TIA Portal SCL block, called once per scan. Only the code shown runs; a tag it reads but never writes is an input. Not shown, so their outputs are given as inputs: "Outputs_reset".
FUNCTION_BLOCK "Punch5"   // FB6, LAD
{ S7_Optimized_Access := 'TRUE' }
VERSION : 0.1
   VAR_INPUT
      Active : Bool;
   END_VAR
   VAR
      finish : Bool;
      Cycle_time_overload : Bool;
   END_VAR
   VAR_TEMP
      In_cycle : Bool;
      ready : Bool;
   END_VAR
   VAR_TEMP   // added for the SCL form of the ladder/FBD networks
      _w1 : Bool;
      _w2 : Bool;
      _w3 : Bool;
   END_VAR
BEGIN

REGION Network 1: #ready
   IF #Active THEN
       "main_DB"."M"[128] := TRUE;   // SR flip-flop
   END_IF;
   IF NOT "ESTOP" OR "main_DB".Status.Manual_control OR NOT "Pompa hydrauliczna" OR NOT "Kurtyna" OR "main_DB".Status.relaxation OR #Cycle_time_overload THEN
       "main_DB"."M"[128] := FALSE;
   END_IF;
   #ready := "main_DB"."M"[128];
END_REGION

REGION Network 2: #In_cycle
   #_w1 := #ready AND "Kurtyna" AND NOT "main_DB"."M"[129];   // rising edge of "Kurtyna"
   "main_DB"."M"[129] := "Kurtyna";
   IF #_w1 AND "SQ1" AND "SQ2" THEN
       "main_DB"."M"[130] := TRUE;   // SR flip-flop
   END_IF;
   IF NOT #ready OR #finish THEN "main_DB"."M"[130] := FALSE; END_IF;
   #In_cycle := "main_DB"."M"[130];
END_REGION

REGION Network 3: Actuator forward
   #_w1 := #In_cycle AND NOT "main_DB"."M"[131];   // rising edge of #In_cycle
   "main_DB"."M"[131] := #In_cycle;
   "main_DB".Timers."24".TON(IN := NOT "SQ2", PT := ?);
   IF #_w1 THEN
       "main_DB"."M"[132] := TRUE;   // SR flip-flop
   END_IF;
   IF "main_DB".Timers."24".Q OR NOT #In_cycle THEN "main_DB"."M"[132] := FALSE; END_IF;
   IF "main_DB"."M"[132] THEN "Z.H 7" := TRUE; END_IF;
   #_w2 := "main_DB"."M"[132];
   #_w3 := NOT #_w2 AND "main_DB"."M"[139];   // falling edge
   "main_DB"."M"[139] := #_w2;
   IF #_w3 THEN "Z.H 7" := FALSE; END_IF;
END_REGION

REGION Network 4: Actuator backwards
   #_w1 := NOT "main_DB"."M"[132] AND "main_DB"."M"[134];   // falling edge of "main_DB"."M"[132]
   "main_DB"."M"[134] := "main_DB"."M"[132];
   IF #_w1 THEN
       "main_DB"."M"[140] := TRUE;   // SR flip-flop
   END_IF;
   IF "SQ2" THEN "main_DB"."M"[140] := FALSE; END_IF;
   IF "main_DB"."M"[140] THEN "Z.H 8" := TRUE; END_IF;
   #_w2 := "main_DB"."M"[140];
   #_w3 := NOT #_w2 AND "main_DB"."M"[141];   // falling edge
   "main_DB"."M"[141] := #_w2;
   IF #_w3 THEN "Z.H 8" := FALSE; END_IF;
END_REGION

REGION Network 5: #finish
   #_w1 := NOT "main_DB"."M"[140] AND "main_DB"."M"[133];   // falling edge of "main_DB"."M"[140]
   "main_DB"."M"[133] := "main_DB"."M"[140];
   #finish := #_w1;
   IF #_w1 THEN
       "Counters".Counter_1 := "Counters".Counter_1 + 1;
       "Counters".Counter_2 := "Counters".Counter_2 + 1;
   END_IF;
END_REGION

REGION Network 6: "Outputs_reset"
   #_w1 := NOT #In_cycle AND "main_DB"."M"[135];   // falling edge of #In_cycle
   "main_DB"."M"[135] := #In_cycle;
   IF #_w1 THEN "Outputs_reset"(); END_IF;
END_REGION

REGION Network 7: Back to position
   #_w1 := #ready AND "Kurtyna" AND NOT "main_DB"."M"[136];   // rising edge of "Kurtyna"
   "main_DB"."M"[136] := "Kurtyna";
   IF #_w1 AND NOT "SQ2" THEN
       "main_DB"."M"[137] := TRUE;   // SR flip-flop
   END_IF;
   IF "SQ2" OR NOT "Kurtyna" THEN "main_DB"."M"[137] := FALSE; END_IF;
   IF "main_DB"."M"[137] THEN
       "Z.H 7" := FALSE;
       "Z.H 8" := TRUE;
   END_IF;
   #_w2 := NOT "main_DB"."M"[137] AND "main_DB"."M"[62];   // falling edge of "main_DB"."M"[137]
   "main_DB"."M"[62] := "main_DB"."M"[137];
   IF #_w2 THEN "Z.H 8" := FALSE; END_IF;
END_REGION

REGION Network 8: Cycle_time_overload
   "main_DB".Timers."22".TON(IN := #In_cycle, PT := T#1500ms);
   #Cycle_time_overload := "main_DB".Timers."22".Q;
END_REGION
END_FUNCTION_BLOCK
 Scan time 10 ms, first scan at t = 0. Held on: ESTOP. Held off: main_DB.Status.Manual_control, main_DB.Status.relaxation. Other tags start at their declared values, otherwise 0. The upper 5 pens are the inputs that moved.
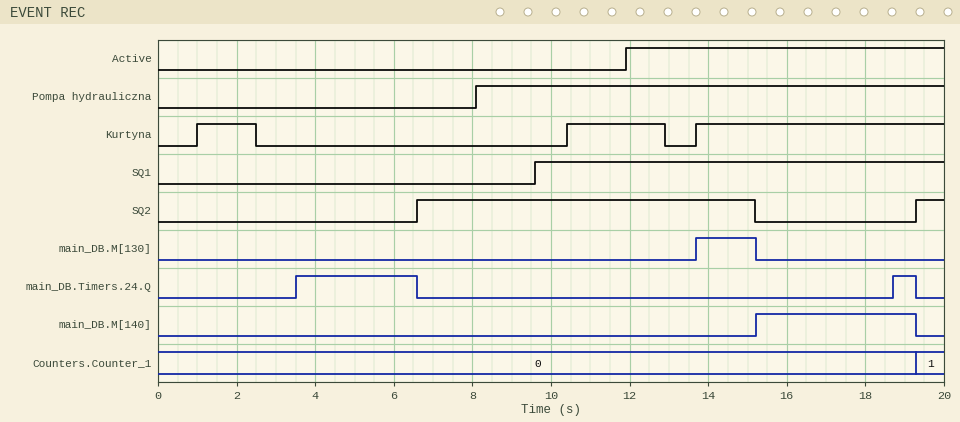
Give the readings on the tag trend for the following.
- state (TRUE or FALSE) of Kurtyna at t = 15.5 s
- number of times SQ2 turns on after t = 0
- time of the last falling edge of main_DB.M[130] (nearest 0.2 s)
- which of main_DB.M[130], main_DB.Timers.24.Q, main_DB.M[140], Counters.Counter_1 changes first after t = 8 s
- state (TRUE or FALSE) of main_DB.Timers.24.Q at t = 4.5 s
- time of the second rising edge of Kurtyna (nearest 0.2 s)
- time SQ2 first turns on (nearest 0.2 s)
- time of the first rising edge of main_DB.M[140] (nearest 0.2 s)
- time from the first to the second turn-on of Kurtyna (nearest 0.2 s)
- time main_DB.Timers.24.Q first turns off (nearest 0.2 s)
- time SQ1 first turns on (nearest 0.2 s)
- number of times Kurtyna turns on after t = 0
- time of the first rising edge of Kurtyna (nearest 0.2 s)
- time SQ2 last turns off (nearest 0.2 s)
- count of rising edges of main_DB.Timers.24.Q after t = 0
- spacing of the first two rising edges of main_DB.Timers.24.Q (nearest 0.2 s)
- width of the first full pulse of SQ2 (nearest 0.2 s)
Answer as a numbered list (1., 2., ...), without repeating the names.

1. TRUE
2. 2
3. 15.2 s
4. main_DB.M[130]
5. TRUE
6. 10.4 s
7. 6.6 s
8. 15.2 s
9. 9.4 s
10. 6.6 s
11. 9.6 s
12. 3
13. 1.0 s
14. 15.2 s
15. 2
16. 15.2 s
17. 8.6 s
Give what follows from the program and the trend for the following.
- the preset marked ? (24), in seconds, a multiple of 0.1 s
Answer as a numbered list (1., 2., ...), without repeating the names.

1. 3.5 s
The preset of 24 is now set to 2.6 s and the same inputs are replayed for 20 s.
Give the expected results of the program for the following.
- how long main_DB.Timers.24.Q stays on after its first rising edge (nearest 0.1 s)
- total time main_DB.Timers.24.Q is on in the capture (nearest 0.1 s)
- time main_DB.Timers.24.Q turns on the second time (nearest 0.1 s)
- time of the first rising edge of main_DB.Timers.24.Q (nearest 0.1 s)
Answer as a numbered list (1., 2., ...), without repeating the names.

1. 4.0 s
2. 5.5 s
3. 17.8 s
4. 2.6 s
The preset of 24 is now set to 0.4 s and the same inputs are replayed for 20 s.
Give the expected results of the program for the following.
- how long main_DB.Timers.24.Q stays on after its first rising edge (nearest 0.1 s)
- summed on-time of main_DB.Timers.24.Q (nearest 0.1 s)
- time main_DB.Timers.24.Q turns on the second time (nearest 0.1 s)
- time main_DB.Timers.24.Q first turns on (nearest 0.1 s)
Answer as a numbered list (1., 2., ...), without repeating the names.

1. 6.2 s
2. 9.9 s
3. 15.6 s
4. 0.4 s
